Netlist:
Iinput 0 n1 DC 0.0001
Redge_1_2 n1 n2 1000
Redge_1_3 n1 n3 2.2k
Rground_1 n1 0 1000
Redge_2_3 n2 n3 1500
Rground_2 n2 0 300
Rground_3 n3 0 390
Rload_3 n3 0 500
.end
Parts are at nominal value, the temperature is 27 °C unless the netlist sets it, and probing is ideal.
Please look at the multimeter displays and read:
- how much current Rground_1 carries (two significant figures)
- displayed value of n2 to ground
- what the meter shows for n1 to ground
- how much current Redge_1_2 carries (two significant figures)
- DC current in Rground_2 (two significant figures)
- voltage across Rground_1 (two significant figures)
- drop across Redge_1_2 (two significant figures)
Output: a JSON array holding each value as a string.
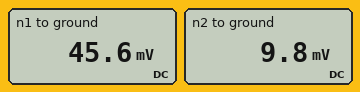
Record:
["46 µA", "9.8 mV", "45.6 mV", "36 µA", "33 µA", "46 mV", "36 mV"]
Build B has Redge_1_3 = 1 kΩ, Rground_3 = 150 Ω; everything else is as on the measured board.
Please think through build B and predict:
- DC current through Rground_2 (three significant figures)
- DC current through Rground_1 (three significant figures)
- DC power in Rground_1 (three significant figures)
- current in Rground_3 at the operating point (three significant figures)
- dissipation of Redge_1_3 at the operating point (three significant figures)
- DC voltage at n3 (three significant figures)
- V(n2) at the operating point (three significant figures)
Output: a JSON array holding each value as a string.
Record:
["26.8 µA", "37.4 µA", "1.40 µW", "27.6 µA", "1.11 µW", "4.14 mV", "8.03 mV"]
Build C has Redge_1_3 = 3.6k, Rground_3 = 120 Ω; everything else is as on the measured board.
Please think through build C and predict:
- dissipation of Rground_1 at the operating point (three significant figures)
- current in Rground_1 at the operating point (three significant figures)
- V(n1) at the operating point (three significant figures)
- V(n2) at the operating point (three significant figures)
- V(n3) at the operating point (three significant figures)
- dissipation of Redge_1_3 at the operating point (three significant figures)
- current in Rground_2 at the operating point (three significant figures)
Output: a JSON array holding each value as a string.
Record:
["2.35 µW", "48.5 µA", "48.5 mV", "9.93 mV", "1.78 mV", "606 nW", "33.1 µA"]
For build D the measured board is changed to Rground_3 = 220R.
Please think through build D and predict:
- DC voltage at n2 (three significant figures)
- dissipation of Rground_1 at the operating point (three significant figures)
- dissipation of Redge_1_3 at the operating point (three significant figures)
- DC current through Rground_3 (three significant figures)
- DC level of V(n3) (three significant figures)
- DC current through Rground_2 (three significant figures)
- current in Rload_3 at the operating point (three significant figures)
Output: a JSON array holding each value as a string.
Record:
["9.52 mV", "2.05 µW", "793 nW", "16.0 µA", "3.51 mV", "31.7 µA", "7.02 µA"]
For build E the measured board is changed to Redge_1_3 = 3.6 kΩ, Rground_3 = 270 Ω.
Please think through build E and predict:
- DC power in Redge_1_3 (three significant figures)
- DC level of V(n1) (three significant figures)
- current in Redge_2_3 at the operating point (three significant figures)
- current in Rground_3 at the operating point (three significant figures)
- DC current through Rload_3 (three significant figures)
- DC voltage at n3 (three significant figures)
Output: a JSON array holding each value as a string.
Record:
["580 nW", "48.7 mV", "4.73 µA", "11.3 µA", "6.11 µA", "3.05 mV"]
